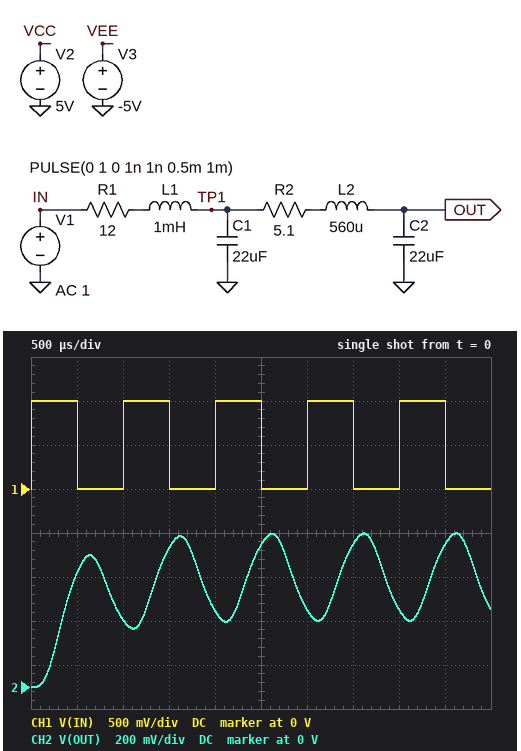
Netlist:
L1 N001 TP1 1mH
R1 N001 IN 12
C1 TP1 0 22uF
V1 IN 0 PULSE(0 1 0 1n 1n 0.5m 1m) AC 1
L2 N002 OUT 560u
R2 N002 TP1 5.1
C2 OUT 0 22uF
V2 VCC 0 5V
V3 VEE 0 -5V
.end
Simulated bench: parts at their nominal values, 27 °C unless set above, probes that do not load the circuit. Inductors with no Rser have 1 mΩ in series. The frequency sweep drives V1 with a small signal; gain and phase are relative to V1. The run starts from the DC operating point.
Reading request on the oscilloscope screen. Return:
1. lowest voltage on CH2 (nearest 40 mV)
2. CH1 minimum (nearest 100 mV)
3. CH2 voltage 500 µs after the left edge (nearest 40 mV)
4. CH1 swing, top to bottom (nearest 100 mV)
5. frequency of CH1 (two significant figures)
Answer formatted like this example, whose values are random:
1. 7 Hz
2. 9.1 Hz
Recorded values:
1. 0 V
2. 0 V
3. 520 mV
4. 1.0 V
5. 1.0 kHz
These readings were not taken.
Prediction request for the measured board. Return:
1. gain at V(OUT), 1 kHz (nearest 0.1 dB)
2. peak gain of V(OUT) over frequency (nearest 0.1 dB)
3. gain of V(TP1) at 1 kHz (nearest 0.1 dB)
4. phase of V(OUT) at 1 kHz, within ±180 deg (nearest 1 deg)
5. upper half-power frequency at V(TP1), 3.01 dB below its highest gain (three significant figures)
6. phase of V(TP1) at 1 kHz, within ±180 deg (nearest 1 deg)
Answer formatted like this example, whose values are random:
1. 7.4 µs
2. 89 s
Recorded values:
1. -10.3 dB
2. 0 dB
3. -11.5 dB
4. -127 deg
5. 310 Hz
6. -73 deg
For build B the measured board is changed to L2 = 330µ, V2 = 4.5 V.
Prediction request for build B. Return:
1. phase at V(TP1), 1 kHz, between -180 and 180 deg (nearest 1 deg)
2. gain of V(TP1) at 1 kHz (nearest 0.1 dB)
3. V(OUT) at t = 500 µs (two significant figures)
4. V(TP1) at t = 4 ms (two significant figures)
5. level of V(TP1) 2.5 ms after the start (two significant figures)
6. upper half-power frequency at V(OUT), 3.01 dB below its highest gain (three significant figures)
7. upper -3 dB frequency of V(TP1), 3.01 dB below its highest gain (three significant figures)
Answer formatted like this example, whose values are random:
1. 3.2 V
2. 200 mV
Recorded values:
1. -79 deg
2. -10.9 dB
3. 510 mV
4. 290 mV
5. 710 mV
6. 316 Hz
7. 314 Hz
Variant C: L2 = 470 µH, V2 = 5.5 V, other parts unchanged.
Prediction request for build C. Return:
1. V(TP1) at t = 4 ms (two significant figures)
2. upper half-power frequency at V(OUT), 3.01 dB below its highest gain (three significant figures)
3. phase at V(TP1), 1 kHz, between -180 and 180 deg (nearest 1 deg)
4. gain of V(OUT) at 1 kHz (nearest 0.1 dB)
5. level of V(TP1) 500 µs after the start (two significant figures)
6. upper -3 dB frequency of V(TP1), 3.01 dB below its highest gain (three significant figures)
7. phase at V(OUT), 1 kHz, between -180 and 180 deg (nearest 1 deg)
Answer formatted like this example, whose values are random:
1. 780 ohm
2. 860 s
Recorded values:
1. 300 mV
2. 321 Hz
3. -76 deg
4. -10.5 dB
5. 590 mV
6. 312 Hz
7. -126 deg
